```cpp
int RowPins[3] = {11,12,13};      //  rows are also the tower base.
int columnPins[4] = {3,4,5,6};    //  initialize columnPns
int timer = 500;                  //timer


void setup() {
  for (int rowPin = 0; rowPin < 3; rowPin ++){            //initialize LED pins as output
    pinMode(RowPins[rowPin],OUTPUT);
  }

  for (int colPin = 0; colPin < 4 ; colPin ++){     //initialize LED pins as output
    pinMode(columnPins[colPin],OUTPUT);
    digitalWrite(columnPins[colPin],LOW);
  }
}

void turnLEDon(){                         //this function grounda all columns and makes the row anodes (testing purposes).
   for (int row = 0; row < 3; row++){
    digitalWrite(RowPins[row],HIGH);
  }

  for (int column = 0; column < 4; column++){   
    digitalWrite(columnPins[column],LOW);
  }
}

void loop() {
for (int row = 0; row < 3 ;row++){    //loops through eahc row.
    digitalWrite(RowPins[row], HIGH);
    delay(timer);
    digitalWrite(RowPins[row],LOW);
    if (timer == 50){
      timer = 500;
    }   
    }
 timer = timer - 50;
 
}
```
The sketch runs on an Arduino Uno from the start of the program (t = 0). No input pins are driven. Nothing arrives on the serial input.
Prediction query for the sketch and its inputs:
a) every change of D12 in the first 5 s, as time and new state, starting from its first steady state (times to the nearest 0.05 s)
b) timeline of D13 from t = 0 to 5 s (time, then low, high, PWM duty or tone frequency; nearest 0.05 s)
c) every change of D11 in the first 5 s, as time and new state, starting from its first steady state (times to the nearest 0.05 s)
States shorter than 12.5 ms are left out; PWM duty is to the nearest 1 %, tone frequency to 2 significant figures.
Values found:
0 s low; 0.5 s high; 1 s low; 1.95 s high; 2.4 s low; 3.25 s high; 3.65 s low; 4.4 s high; 4.75 s low
0 s low; 1 s high; 1.5 s low; 2.4 s high; 2.85 s low; 3.65 s high; 4.05 s low; 4.75 s high
0 s high; 0.5 s low; 1.5 s high; 1.95 s low; 2.85 s high; 3.25 s low; 4.05 s high; 4.4 s low
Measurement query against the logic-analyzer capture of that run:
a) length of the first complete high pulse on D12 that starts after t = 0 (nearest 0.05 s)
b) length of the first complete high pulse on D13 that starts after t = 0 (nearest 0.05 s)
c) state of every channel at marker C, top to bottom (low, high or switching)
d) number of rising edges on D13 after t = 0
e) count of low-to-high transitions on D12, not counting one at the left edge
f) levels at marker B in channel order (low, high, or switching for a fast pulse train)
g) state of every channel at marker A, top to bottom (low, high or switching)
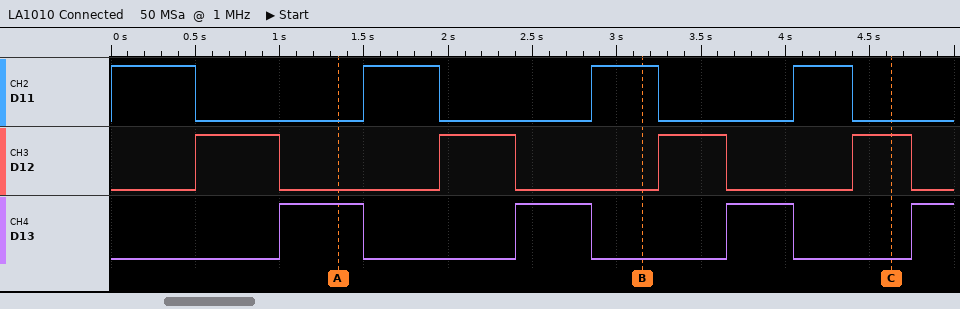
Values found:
0.50 s
0.50 s
D11 low, D12 high, D13 low
4
4
D11 high, D12 low, D13 low
D11 low, D12 low, D13 high
